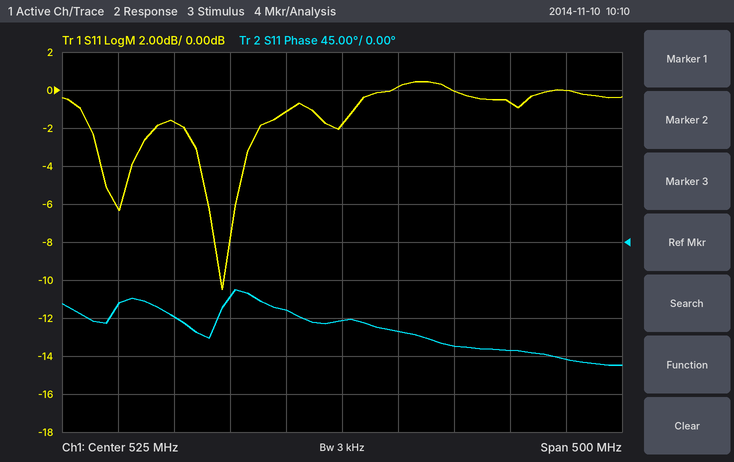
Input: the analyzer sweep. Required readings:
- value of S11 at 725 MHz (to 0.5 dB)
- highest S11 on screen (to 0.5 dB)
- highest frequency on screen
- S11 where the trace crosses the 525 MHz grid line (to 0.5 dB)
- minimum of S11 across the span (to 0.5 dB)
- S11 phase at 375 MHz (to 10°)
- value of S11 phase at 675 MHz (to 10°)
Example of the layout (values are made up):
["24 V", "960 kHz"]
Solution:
["0.0 dB", "0.5 dB", "775 MHz", "-2.0 dB", "-10.5 dB", "-90°", "-130°"]
